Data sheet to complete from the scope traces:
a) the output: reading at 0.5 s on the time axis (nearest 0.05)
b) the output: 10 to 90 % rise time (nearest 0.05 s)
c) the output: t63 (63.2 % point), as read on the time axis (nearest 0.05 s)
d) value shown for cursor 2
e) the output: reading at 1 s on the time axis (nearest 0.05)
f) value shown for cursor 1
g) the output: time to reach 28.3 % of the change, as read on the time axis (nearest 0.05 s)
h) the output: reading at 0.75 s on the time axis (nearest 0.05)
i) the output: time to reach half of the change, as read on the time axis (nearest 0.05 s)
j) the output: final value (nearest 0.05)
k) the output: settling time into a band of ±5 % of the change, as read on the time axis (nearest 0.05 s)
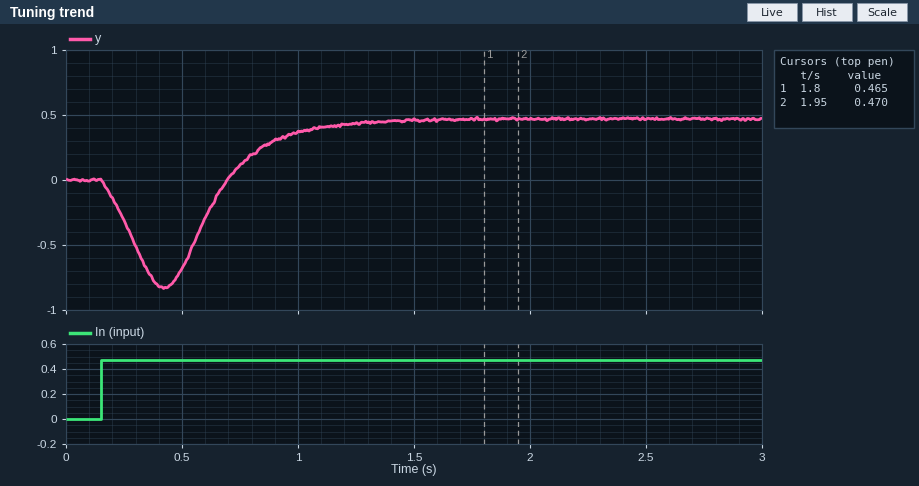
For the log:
-0.70
0.45 s
0.90 s
0.470
0.35
0.465
0.75 s
0.10
0.85 s
0.45
1.35 s
